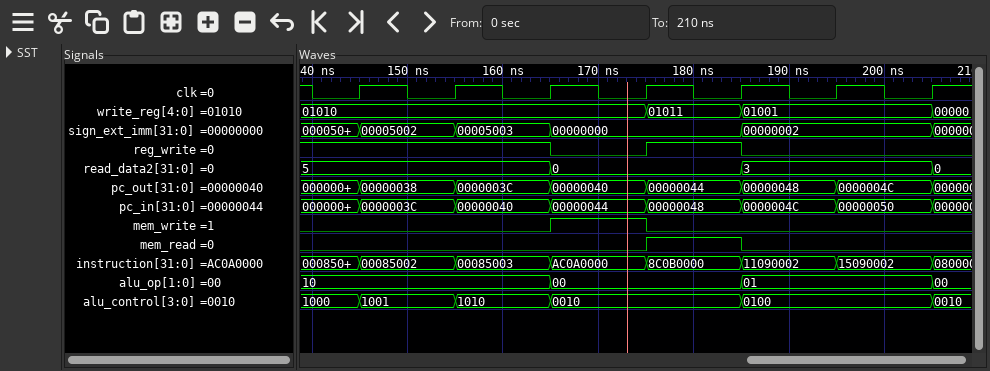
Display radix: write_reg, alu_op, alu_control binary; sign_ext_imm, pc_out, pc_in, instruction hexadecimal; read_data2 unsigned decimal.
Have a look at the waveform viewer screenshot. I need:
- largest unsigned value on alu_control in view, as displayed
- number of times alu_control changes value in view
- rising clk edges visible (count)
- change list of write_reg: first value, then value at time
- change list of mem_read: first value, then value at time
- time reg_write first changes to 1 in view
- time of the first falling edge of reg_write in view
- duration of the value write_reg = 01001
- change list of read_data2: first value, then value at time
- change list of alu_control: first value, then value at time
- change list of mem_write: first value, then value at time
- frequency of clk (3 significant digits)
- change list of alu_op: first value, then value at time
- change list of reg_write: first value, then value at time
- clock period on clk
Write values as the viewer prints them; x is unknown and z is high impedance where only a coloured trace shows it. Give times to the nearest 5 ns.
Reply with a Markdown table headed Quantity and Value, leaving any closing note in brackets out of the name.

| Quantity | Value |
|---|---|
| largest unsigned value on alu_control in view, as displayed | 1010 |
| number of times alu_control changes value in view | 5 |
| rising clk edges visible | 7 |
| change list of write_reg: first value, then value at time | 01010, 01011 at 175 ns, 01001 at 185 ns, 00000 at 205 ns |
| change list of mem_read: first value, then value at time | 0, 1 at 175 ns, 0 at 185 ns |
| time reg_write first changes to 1 in view | 175 ns |
| time of the first falling edge of reg_write in view | 165 ns |
| duration of the value write_reg = 01001 | 20 ns |
| change list of read_data2: first value, then value at time | 5, 0 at 165 ns, 3 at 185 ns, 0 at 205 ns |
| change list of alu_control: first value, then value at time | 1000, 1001 at 145 ns, 1010 at 155 ns, 0010 at 165 ns, 0100 at 185 ns, 0010 at 205 ns |
| change list of mem_write: first value, then value at time | 0, 1 at 165 ns, 0 at 175 ns |
| frequency of clk | 100 MHz |
| change list of alu_op: first value, then value at time | 10, 00 at 165 ns, 01 at 185 ns, 00 at 205 ns |
| change list of reg_write: first value, then value at time | 1, 0 at 165 ns, 1 at 175 ns, 0 at 185 ns |
| clock period on clk | 10 ns |
